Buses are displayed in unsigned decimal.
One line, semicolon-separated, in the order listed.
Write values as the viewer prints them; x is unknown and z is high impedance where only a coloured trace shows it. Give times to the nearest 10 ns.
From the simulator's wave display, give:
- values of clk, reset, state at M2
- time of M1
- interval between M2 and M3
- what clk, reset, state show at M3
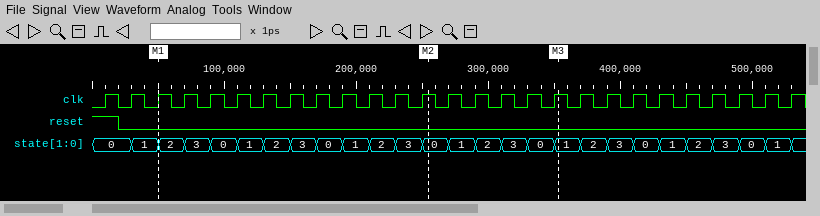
clk=1, reset=0, state=0; 50 ns; 100 ns; clk=1, reset=0, state=1
